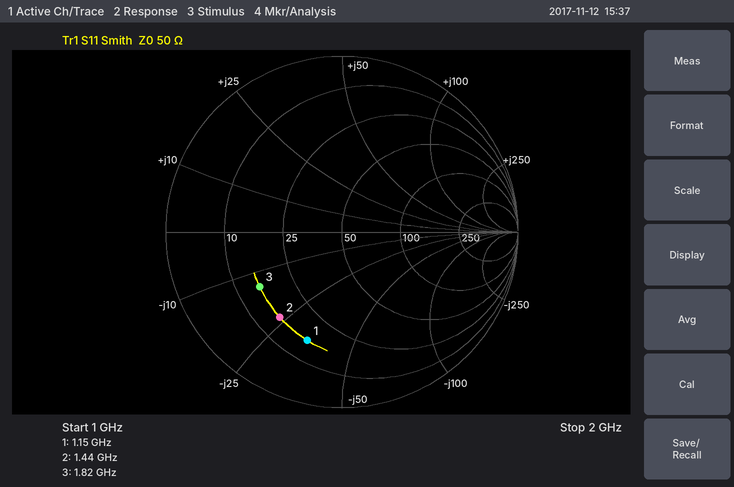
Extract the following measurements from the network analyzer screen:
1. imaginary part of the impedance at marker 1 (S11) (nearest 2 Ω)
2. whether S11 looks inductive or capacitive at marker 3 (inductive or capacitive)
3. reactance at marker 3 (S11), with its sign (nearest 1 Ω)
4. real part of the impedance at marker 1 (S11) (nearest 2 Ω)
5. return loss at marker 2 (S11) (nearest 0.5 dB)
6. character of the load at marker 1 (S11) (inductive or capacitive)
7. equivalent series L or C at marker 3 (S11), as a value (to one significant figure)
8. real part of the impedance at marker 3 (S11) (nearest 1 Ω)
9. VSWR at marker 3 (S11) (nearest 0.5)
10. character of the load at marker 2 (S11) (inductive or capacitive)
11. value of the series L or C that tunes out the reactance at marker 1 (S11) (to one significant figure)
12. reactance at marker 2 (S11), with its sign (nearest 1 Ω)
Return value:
-34 Ω
capacitive
-14 Ω
16 Ω
4.5 dB
capacitive
6 pF
15 Ω
3.5
capacitive
5 nH
-23 Ω
